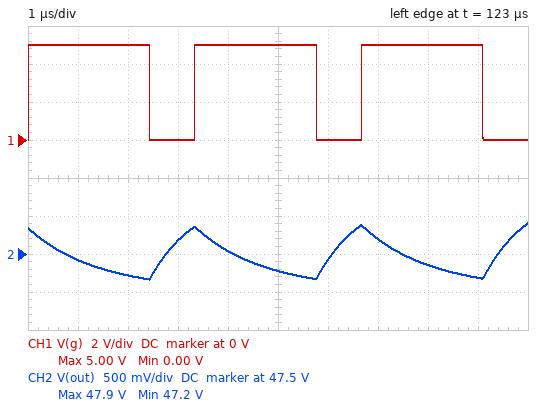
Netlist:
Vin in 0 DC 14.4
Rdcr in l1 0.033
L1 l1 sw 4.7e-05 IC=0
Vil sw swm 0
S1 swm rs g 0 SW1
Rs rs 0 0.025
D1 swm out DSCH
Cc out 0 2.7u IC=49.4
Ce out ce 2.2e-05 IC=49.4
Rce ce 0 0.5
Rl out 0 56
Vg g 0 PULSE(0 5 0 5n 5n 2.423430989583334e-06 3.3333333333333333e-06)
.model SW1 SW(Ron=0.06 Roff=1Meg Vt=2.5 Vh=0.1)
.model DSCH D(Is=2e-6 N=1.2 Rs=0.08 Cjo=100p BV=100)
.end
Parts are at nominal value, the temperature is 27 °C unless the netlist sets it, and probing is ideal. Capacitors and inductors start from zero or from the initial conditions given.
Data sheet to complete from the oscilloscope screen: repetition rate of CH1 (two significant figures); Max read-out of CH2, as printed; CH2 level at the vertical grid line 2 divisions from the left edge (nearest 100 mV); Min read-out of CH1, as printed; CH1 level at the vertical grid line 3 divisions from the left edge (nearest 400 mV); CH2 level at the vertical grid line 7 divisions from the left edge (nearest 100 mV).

300 kHz
47.9 V
47.2 V
0.00 V
0 V
47.7 V
